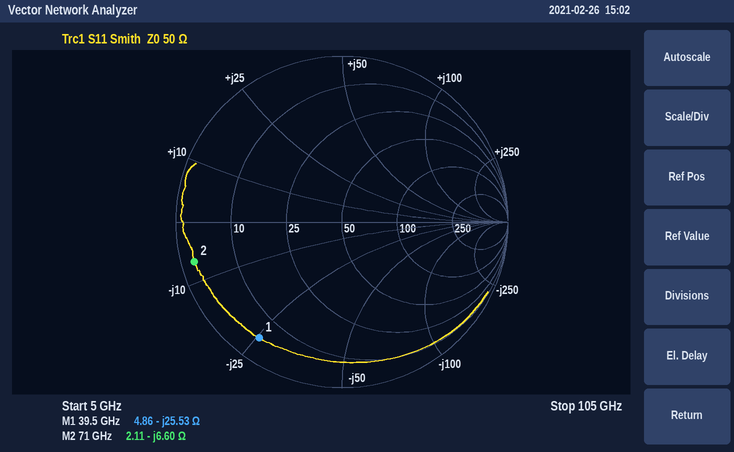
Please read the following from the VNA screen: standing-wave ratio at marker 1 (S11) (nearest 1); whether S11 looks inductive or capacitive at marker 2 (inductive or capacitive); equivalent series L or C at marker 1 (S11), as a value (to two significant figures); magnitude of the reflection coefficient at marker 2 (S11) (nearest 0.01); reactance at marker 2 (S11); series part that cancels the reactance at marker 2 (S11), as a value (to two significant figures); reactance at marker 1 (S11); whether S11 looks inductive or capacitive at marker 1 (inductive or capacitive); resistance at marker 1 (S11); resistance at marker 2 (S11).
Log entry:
13
capacitive
160 fF
0.92
-6.60 Ω
15 pH
-25.53 Ω
capacitive
4.86 Ω
2.11 Ω
